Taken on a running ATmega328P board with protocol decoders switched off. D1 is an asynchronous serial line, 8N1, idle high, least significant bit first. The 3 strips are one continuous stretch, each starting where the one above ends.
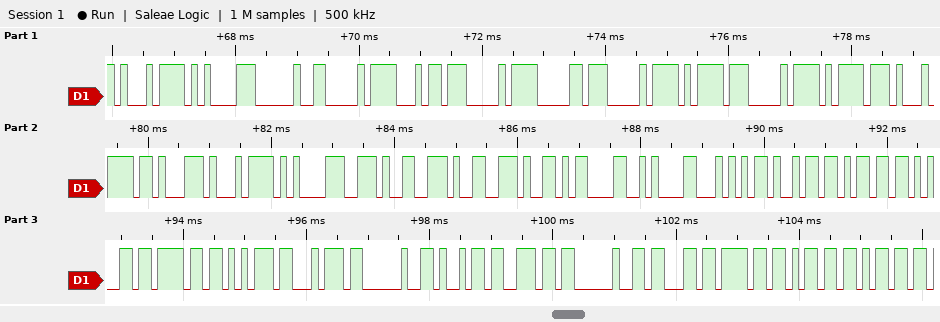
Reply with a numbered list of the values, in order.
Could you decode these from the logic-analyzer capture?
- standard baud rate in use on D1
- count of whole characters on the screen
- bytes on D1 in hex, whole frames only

1. 9600 baud
2. 35
3. D1 85 20 D0 B4 D0 B0 D0 BD D0 BD D1 8B D1 85 2E 2E 2E 0D 0A 54 69 6D 65 6F 75 74 20 69 6E 20 63 6F 6D 6D
